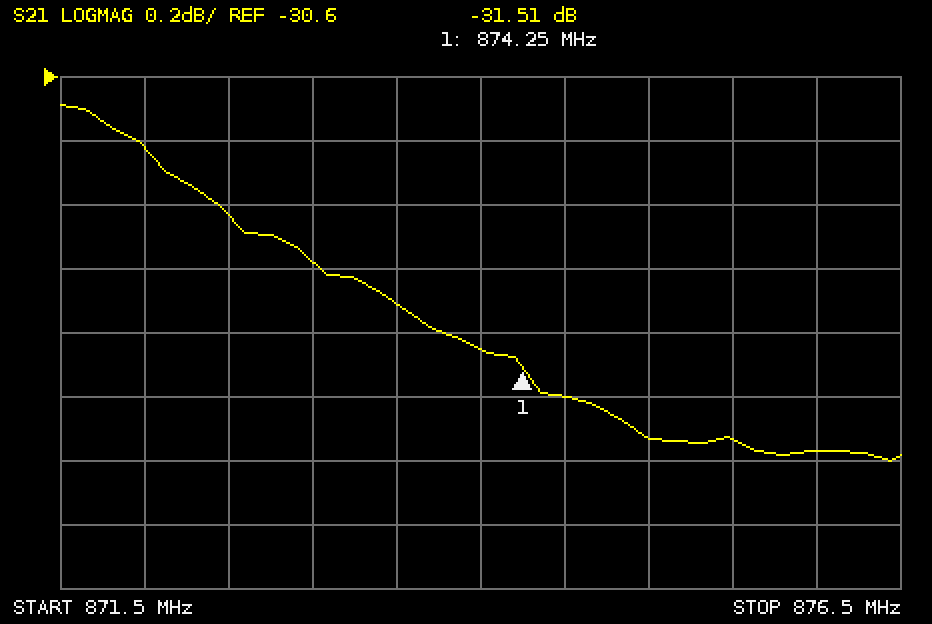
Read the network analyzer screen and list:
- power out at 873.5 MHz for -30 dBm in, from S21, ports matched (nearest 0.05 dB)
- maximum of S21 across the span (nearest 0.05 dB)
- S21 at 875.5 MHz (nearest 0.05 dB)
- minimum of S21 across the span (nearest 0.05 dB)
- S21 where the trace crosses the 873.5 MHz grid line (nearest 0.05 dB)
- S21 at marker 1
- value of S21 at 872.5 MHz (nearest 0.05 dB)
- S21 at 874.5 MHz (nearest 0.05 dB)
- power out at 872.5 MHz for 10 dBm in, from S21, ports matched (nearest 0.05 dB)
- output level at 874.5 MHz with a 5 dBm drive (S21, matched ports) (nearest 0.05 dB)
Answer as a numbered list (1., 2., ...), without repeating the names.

1. -61.30 dBm
2. -30.70 dB
3. -31.75 dB
4. -31.80 dB
5. -31.30 dB
6. -31.51 dB
7. -31.05 dB
8. -31.60 dB
9. -21.05 dBm
10. -26.60 dBm
